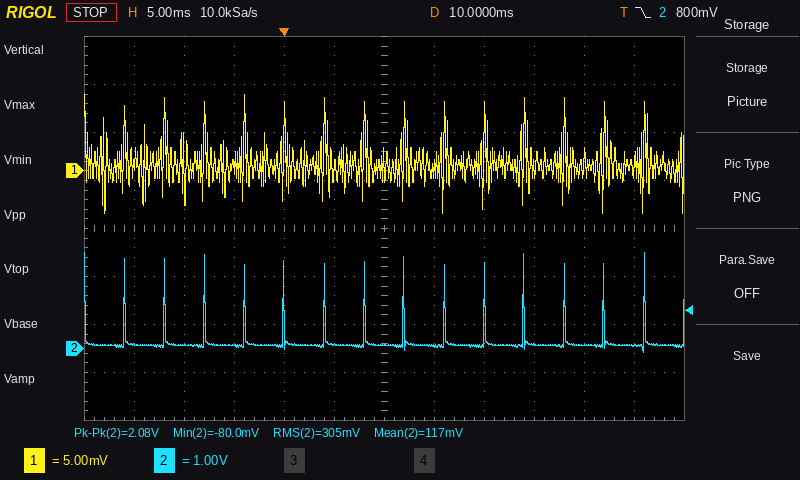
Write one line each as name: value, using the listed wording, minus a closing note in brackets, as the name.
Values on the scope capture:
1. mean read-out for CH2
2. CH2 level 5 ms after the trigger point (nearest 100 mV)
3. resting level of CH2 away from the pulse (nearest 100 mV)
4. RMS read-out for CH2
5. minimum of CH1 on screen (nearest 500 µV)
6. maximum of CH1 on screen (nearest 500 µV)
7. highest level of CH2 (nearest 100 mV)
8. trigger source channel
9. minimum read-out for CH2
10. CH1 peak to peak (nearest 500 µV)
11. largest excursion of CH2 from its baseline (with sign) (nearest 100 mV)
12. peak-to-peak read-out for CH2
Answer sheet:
mean read-out for CH2: 117 mV
CH2 level 5 ms after the trigger point: 100 mV
resting level of CH2 away from the pulse: 100 mV
RMS read-out for CH2: 305 mV
minimum of CH1 on screen: -4.5 mV
maximum of CH1 on screen: 8.0 mV
highest level of CH2: 2.0 V
trigger source channel: CH2
minimum read-out for CH2: -80.0 mV
CH1 peak to peak: 12.5 mV
largest excursion of CH2 from its baseline (with sign): +1.9 V
peak-to-peak read-out for CH2: 2.08 V
